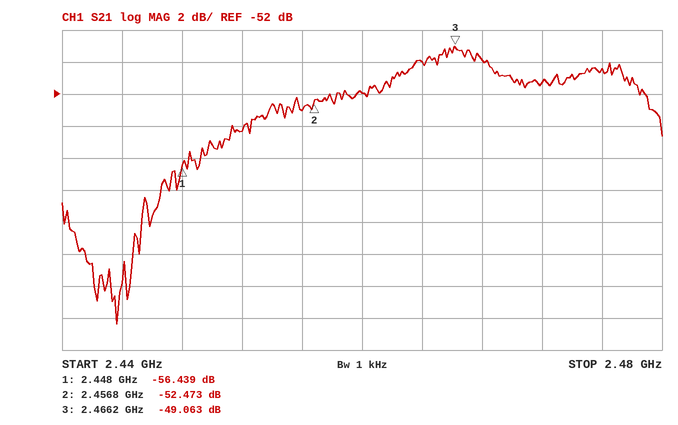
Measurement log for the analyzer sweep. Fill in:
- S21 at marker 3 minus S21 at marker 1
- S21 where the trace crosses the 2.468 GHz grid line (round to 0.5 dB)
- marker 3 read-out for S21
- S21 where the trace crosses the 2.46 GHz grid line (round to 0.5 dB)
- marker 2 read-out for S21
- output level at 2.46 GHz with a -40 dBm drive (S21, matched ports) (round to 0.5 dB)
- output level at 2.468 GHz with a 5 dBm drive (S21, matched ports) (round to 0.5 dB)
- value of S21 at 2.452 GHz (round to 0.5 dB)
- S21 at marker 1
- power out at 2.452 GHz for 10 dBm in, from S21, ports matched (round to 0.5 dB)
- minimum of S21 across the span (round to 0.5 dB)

7.376 dB
-50.0 dB
-49.063 dB
-52.0 dB
-52.473 dB
-92.0 dBm
-45.0 dBm
-54.5 dB
-56.439 dB
-44.5 dBm
-66.5 dB
